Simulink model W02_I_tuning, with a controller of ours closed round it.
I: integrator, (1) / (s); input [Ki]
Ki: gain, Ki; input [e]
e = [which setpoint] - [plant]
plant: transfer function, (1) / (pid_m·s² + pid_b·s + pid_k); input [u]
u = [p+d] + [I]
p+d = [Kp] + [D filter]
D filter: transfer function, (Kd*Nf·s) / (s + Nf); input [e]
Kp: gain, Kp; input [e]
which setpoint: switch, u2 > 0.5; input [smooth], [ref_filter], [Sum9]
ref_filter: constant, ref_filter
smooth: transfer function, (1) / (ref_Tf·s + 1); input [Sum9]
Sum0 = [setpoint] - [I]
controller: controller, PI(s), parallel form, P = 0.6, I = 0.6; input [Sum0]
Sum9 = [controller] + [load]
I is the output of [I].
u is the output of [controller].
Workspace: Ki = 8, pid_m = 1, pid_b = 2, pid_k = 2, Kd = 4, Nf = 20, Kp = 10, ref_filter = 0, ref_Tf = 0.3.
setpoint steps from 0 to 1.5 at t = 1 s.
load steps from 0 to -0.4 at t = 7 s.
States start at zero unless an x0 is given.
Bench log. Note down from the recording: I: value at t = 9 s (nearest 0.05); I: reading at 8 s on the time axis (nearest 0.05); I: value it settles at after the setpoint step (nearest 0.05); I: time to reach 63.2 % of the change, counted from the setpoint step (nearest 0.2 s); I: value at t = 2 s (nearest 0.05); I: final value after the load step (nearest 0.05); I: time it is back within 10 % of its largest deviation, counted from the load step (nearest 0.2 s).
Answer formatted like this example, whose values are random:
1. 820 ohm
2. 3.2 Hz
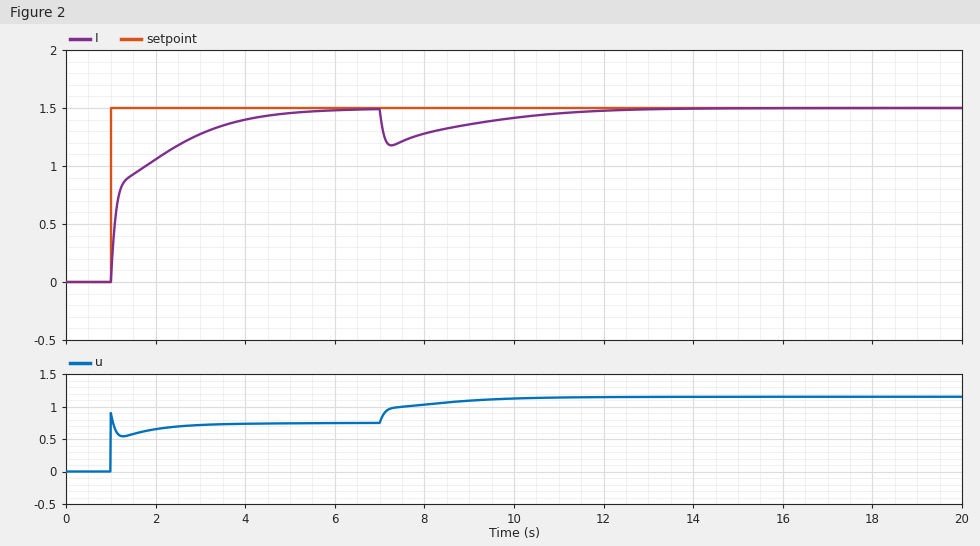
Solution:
1. 1.35
2. 1.30
3. 1.50
4. 0.6 s
5. 1.05
6. 1.50
7. 4.6 s
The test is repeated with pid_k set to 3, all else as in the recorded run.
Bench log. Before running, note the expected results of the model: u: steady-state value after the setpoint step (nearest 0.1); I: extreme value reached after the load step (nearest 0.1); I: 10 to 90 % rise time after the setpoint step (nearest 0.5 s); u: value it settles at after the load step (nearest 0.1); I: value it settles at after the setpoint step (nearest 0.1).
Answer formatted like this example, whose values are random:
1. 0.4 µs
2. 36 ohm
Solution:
1. 0.5
2. 1.2
3. 1.5 s
4. 0.9
5. 1.5
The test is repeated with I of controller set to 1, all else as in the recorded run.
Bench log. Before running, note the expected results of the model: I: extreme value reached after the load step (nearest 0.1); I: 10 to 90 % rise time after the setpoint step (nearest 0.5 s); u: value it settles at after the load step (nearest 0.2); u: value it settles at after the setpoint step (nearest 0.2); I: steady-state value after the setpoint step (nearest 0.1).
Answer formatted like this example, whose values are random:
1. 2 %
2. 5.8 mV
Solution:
1. 1.2
2. 1.5 s
3. 1.2
4. 0.8
5. 1.5
